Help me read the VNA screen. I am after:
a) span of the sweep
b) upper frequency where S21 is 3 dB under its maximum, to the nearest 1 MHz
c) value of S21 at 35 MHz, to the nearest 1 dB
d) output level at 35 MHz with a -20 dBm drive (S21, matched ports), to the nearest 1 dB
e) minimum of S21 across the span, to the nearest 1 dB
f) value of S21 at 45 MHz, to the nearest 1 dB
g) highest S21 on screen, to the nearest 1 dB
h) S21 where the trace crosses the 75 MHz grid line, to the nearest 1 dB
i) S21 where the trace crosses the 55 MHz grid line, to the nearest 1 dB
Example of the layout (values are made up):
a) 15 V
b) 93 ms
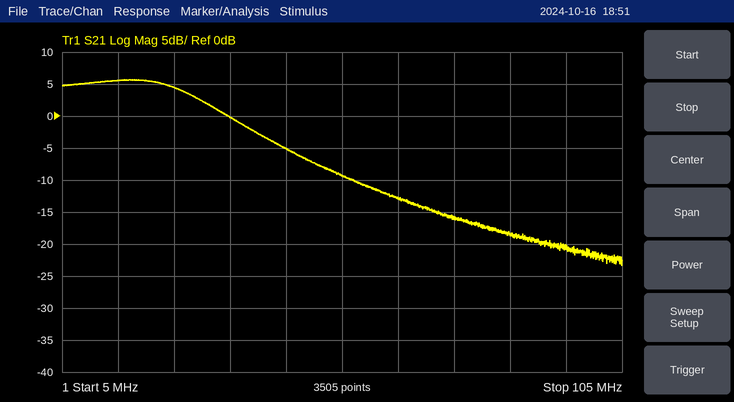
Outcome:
a) 100 MHz
b) 29 MHz
c) 0 dB
d) -20 dBm
e) -23 dB
f) -5 dB
g) 6 dB
h) -16 dB
i) -9 dB
